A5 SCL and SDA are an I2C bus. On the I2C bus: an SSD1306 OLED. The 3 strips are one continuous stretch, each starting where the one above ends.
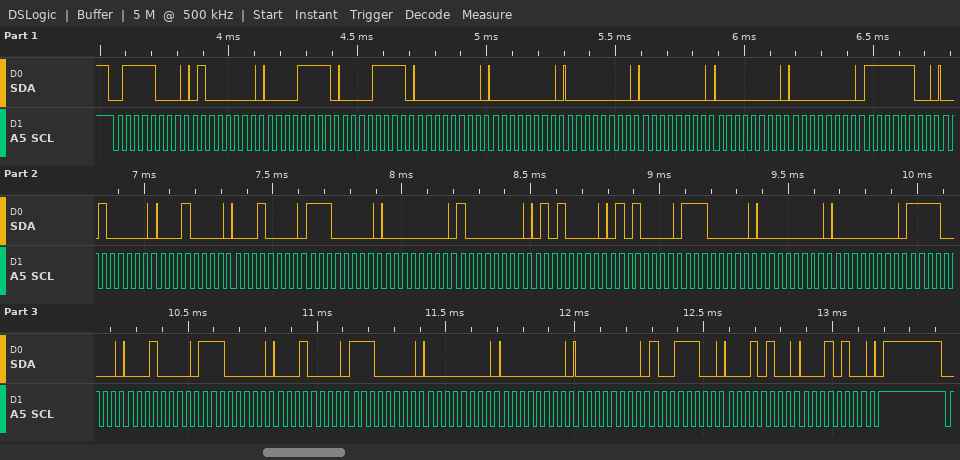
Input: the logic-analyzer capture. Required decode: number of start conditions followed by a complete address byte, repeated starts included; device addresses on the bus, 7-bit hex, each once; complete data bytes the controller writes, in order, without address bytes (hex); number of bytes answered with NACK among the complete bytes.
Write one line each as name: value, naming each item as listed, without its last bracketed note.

number of start conditions followed by a complete address byte, repeated starts included: 1
device addresses on the bus, 7-bit hex, each once: 0x3C
complete data bytes the controller writes, in order, without address bytes: 40 0F 0F 00 00 00 00 00 00 FC 20 10 10 E0 00 80 50 50 E0 00 00 F0 10 E0 10 E0 00 00 00 9C 14 14
number of bytes answered with NACK among the complete bytes: 0
